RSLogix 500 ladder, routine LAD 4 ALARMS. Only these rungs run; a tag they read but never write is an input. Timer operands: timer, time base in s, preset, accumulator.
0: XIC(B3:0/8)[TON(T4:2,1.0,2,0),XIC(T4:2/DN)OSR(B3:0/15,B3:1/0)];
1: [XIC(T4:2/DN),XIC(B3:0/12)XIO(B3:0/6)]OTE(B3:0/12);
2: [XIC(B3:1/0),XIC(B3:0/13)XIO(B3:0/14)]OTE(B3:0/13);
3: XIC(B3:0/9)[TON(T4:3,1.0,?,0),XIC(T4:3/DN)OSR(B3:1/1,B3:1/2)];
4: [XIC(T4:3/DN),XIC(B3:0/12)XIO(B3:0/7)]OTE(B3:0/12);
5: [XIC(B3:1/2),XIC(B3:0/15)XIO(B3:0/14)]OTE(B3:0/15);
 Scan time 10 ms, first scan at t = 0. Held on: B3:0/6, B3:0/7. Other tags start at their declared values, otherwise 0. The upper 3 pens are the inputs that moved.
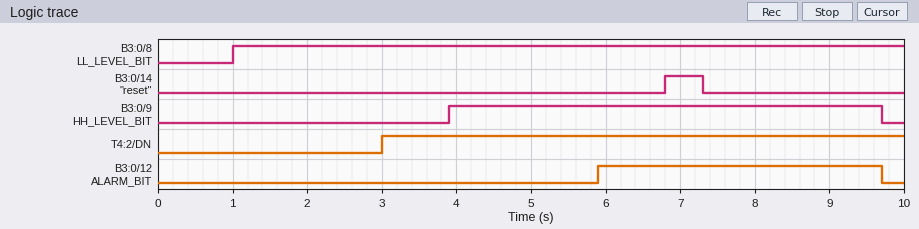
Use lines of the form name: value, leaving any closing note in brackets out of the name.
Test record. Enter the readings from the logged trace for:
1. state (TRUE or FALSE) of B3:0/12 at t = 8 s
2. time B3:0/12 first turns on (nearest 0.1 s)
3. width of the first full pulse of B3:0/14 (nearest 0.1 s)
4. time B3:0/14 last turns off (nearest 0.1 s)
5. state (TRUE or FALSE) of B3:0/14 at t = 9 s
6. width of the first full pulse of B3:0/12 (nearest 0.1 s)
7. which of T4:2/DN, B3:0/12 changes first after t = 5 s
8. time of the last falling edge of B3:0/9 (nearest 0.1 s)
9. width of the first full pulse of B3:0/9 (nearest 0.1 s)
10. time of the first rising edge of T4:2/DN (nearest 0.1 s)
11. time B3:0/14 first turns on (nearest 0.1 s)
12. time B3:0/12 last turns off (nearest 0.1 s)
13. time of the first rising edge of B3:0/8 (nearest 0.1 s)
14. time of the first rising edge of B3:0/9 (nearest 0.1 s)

state (TRUE or FALSE) of B3:0/12 at t = 8 s: TRUE
time B3:0/12 first turns on: 5.9 s
width of the first full pulse of B3:0/14: 0.5 s
time B3:0/14 last turns off: 7.3 s
state (TRUE or FALSE) of B3:0/14 at t = 9 s: FALSE
width of the first full pulse of B3:0/12: 3.8 s
which of T4:2/DN, B3:0/12 changes first after t = 5 s: B3:0/12
time of the last falling edge of B3:0/9: 9.7 s
width of the first full pulse of B3:0/9: 5.8 s
time of the first rising edge of T4:2/DN: 3.0 s
time B3:0/14 first turns on: 6.8 s
time B3:0/12 last turns off: 9.7 s
time of the first rising edge of B3:0/8: 1.0 s
time of the first rising edge of B3:0/9: 3.9 s
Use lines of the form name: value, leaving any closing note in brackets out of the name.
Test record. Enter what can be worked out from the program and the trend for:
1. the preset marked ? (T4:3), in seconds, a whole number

the preset marked ? (T4:3), in seconds, a whole number: 2 s
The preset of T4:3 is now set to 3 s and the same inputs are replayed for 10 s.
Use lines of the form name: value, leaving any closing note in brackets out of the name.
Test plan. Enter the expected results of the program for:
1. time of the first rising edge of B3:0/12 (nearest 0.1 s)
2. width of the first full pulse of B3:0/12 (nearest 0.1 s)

time of the first rising edge of B3:0/12: 6.9 s
width of the first full pulse of B3:0/12: 2.8 s
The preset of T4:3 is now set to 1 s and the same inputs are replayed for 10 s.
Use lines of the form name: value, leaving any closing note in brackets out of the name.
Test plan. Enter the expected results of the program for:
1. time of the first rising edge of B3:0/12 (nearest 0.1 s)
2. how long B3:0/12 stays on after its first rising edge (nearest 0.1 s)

time of the first rising edge of B3:0/12: 4.9 s
how long B3:0/12 stays on after its first rising edge: 4.8 s
